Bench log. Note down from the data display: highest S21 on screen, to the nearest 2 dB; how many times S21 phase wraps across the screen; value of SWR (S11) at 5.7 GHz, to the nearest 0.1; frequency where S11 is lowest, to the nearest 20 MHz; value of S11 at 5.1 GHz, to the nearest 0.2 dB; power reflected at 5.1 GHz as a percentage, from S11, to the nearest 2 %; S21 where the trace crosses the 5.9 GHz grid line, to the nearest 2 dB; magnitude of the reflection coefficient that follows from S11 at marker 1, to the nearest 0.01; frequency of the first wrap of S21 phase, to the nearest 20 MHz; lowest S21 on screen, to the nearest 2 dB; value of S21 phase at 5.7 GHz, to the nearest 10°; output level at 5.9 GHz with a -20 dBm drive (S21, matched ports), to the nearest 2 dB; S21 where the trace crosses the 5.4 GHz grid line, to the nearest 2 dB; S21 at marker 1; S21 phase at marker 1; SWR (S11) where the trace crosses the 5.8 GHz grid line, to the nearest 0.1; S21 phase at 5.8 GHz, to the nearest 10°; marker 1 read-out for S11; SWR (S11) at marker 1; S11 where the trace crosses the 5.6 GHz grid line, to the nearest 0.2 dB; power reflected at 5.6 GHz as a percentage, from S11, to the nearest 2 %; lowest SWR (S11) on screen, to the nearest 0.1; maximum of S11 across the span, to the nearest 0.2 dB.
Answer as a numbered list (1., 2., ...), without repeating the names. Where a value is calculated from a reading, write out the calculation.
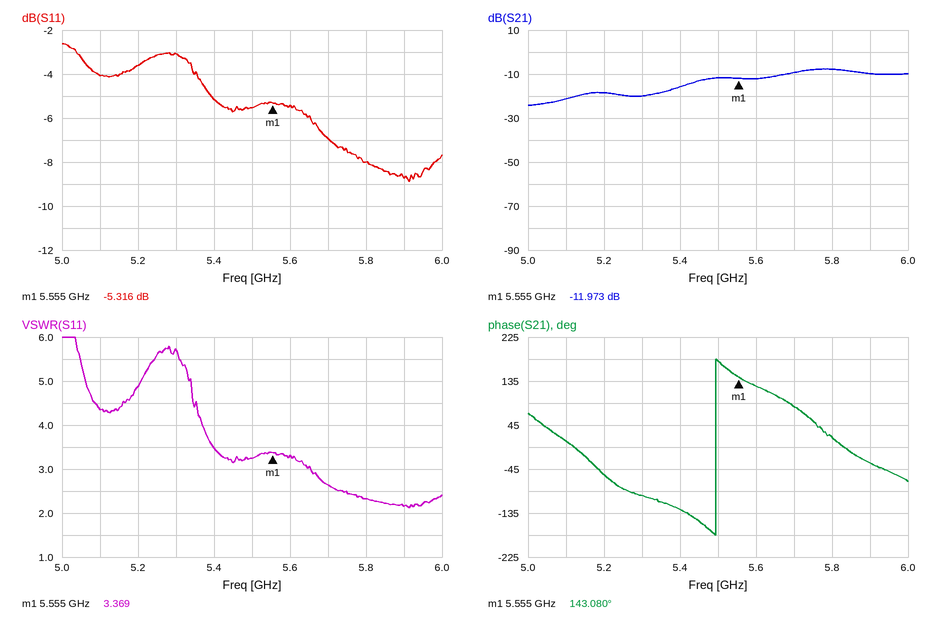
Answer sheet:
1. -8 dB
2. 1
3. 2.6
4. 5.92 GHz
5. -4.0 dB
6. 10^(-4/10) ≈ 40 %
7. -10 dB
8. 10^(-5.316/20) ≈ 0.54
9. 5.50 GHz
10. -24 dB
11. 80°
12. -20 dBm + (-10 dB) = -30 dBm
13. -16 dB
14. -11.973 dB
15. 143.080°
16. 2.3
17. 20°
18. -5.316 dB
19. 3.369
20. -5.4 dB
21. 10^(-5.4/10) ≈ 28.8 %, so 28 % to the nearest 2 %
22. 2.1
23. -2.6 dB
